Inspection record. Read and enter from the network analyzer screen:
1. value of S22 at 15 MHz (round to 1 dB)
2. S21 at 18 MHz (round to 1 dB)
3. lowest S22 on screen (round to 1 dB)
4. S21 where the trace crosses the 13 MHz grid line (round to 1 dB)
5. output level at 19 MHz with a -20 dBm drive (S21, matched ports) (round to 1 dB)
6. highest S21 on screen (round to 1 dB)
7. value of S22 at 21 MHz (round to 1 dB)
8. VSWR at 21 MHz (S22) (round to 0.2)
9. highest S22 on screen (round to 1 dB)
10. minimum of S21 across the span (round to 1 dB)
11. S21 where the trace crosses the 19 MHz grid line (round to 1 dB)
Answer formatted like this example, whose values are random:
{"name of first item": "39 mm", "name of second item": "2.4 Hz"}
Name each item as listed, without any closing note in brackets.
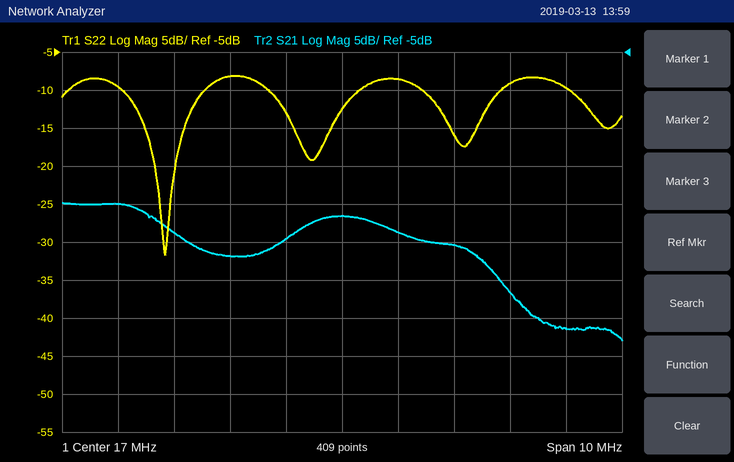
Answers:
{"value of S22 at 15 MHz": "-8 dB", "S21 at 18 MHz": "-29 dB", "lowest S22 on screen": "-32 dB", "S21 where the trace crosses the 13 MHz grid line": "-25 dB", "output level at 19 MHz with a -20 dBm drive (S21, matched ports)": "-50 dBm", "highest S21 on screen": "-25 dB", "value of S22 at 21 MHz": "-10 dB", "VSWR at 21 MHz (S22)": "2.0", "highest S22 on screen": "-8 dB", "minimum of S21 across the span": "-43 dB", "S21 where the trace crosses the 19 MHz grid line": "-30 dB"}
